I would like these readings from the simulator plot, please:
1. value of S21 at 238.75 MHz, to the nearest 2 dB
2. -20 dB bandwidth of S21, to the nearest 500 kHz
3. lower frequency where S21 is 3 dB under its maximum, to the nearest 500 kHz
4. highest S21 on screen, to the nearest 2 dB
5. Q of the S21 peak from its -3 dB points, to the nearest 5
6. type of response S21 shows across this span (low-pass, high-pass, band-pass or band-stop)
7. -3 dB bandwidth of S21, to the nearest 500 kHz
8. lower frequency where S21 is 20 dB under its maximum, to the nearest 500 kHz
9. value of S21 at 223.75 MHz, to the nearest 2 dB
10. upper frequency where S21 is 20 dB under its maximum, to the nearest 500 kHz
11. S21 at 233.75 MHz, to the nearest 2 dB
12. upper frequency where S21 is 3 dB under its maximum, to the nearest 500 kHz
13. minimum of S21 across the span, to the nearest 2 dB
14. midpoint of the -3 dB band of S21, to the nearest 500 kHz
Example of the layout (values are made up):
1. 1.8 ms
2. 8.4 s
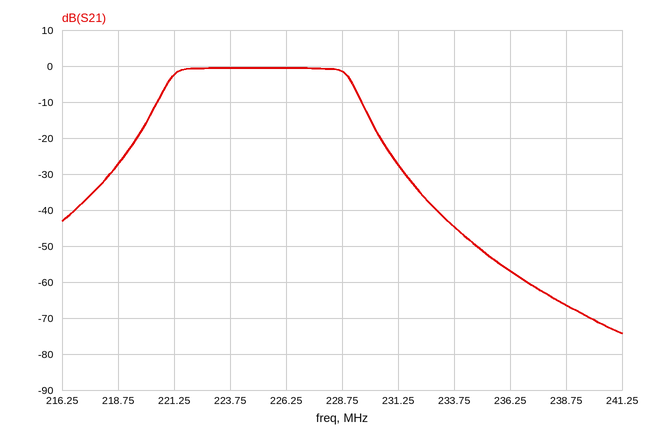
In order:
1. -66 dB
2. 11.0 MHz
3. 221.0 MHz
4. 0 dB
5. 30
6. band-pass
7. 8.0 MHz
8. 219.5 MHz
9. 0 dB
10. 230.5 MHz
11. -44 dB
12. 229.0 MHz
13. -74 dB
14. 225.0 MHz
